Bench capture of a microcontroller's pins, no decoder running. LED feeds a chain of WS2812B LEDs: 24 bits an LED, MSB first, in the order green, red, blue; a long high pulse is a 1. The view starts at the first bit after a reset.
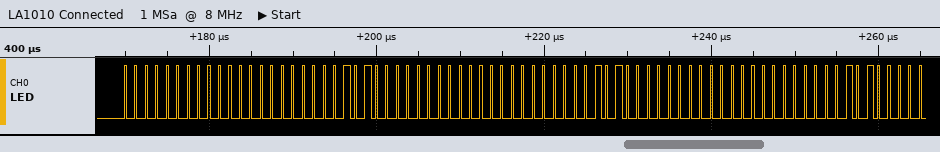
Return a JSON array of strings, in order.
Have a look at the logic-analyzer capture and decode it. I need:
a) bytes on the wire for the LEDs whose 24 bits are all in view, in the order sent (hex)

["00 00 05 00 00 05 00 00 05"]
